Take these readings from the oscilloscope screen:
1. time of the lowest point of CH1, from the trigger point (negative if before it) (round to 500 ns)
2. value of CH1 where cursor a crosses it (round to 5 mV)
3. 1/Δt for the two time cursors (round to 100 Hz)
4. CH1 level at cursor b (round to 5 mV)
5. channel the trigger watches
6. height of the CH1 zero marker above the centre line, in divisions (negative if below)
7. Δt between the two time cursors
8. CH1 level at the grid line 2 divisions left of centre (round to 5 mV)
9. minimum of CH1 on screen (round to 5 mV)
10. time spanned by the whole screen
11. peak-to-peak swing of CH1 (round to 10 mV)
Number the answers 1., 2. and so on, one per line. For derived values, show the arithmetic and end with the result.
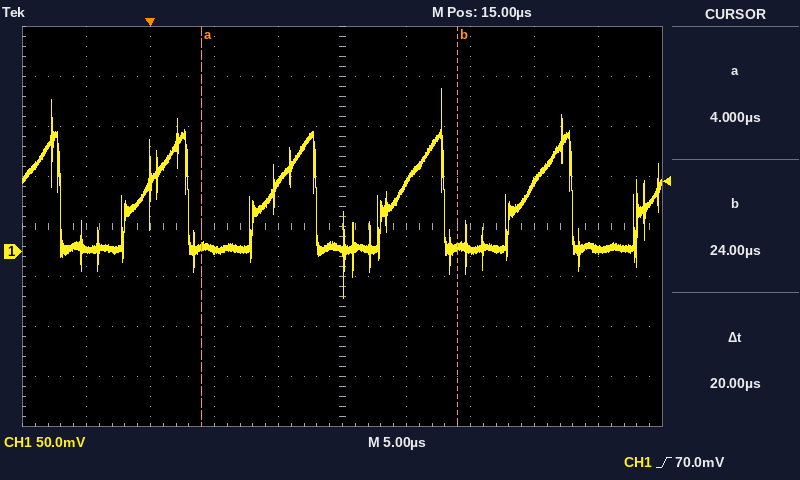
1. +15.0 µs
2. 5 mV
3. 1 / 20 µs ≈ 50.0 kHz
4. 5 mV
5. CH1
6. -0.5 div
7. 20 µs
8. 0 mV
9. -45 mV
10. 50 µs
11. 210 mV
